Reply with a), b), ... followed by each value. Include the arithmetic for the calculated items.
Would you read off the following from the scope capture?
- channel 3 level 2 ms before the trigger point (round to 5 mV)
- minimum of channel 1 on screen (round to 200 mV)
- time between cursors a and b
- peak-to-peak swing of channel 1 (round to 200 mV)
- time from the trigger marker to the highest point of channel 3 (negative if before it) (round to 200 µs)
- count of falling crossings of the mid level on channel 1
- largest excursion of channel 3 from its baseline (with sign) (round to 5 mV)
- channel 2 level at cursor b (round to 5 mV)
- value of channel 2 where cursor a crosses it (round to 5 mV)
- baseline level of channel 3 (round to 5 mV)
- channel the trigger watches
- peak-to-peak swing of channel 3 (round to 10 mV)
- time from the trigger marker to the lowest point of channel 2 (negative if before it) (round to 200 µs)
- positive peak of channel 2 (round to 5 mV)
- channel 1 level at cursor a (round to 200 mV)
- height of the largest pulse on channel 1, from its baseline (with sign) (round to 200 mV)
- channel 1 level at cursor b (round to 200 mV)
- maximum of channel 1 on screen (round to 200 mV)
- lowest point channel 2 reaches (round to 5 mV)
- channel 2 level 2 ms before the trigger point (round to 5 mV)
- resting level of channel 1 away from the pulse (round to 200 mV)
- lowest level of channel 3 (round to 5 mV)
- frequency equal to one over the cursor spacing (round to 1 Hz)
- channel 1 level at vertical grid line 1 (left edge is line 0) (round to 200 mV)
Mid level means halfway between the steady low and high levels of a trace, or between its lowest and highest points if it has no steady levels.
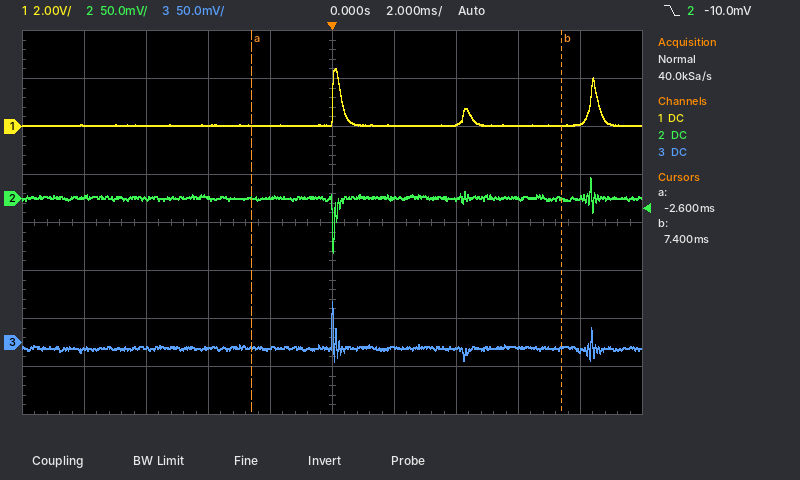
a) -5 mV
b) 0.0 V
c) 7.4 ms − (-2.6 ms) = 10.0 ms
d) 2.4 V − (0.0 V) = 2.4 V
e) 0.0 ms
f) 2
g) +50 mV
h) 0 mV
i) 0 mV
j) -5 mV
k) channel 2
l) 60 mV
m) 0.0 ms
n) 20 mV
o) 0.0 V
p) 2.4 V − (0.0 V) = +2.4 V
q) 0.0 V
r) 2.4 V
s) -55 mV
t) 0 mV
u) 0.0 V
v) -20 mV
w) 1 / 10.0 ms ≈ 100 Hz
x) 0.0 V
